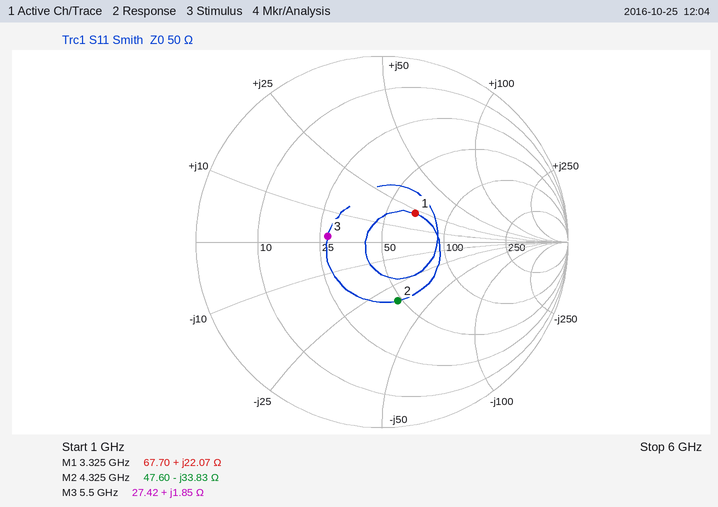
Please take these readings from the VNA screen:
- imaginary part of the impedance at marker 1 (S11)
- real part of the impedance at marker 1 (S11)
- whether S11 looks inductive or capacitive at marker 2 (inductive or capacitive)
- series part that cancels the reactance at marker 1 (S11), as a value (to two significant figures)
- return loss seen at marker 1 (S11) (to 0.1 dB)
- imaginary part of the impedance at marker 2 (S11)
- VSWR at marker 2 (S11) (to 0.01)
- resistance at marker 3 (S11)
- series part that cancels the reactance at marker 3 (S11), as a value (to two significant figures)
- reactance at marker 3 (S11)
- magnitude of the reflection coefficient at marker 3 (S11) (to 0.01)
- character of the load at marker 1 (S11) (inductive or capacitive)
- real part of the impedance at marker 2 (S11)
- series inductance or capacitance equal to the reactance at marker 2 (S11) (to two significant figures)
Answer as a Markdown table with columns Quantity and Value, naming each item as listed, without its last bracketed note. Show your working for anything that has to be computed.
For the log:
| Quantity | Value |
|---|---|
| imaginary part of the impedance at marker 1 | +22.07 Ω |
| real part of the impedance at marker 1 | 67.70 Ω |
| whether S11 looks inductive or capacitive at marker 2 | capacitive |
| series part that cancels the reactance at marker 1 (S11), as a value | C = 1/(2π × 3.325 GHz × 22.07 Ω) ≈ 2.2 pF |
| return loss seen at marker 1 (S11) | 12.5 dB |
| imaginary part of the impedance at marker 2 | -33.83 Ω |
| VSWR at marker 2 (S11) | 1.98 |
| resistance at marker 3 | 27.42 Ω |
| series part that cancels the reactance at marker 3 (S11), as a value | C = 1/(2π × 5.5 GHz × 1.85 Ω) ≈ 16 pF |
| reactance at marker 3 | +1.85 Ω |
| magnitude of the reflection coefficient at marker 3 (S11) | 0.29 |
| character of the load at marker 1 (S11) | inductive |
| real part of the impedance at marker 2 | 47.60 Ω |
| series inductance or capacitance equal to the reactance at marker 2 (S11) | C = 1/(2π × 4.325 GHz × 33.83 Ω) ≈ 1.1 pF |
